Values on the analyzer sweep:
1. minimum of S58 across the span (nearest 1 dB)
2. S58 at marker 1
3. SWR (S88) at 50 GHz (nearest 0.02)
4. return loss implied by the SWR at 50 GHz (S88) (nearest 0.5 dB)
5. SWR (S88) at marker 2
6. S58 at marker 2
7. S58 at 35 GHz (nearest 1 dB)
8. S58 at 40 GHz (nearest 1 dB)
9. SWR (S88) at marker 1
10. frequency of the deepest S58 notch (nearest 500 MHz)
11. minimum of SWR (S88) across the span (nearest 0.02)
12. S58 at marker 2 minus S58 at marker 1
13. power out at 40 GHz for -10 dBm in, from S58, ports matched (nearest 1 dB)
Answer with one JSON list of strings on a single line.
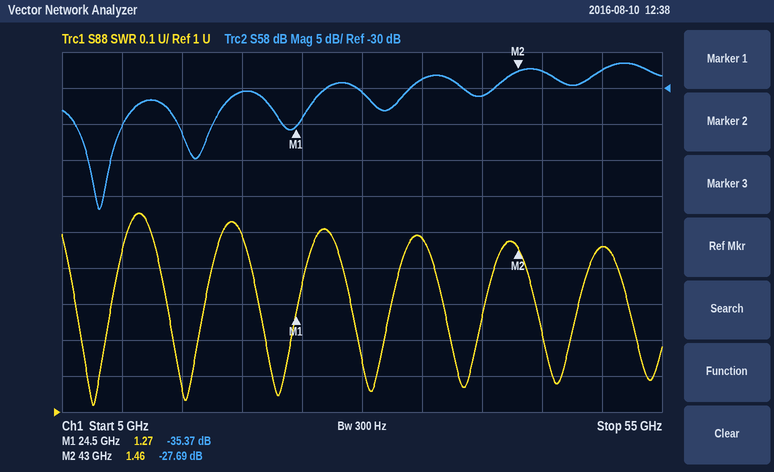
["-47 dB", "-35.37 dB", "1.46", "14.5 dB", "1.46", "-27.69 dB", "-29 dB", "-31 dB", "1.27", "8.0 GHz", "1.02", "7.68 dB", "-41 dBm"]
